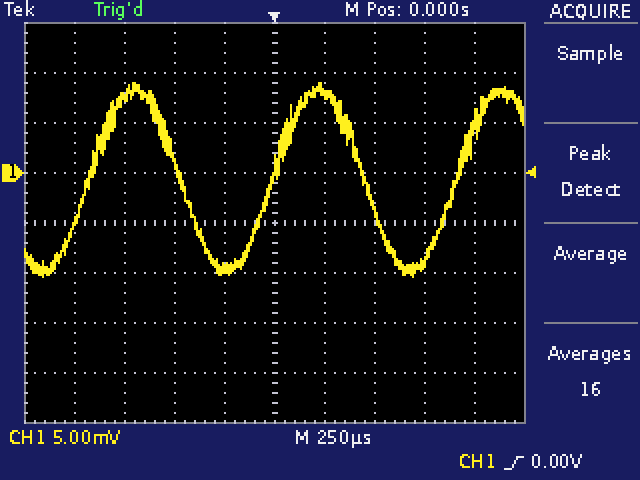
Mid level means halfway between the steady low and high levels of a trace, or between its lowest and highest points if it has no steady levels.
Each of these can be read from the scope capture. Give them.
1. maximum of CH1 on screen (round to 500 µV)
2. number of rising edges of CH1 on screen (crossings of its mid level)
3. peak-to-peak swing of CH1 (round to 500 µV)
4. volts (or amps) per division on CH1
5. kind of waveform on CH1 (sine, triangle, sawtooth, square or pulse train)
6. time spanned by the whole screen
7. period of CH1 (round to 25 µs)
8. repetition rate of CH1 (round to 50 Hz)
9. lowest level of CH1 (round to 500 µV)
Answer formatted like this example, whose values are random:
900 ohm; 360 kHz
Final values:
9.0 mV; 3; 19.5 mV; 5 mV; sine; 2.5 ms; 925 µs; 1.10 kHz; -10.5 mV
